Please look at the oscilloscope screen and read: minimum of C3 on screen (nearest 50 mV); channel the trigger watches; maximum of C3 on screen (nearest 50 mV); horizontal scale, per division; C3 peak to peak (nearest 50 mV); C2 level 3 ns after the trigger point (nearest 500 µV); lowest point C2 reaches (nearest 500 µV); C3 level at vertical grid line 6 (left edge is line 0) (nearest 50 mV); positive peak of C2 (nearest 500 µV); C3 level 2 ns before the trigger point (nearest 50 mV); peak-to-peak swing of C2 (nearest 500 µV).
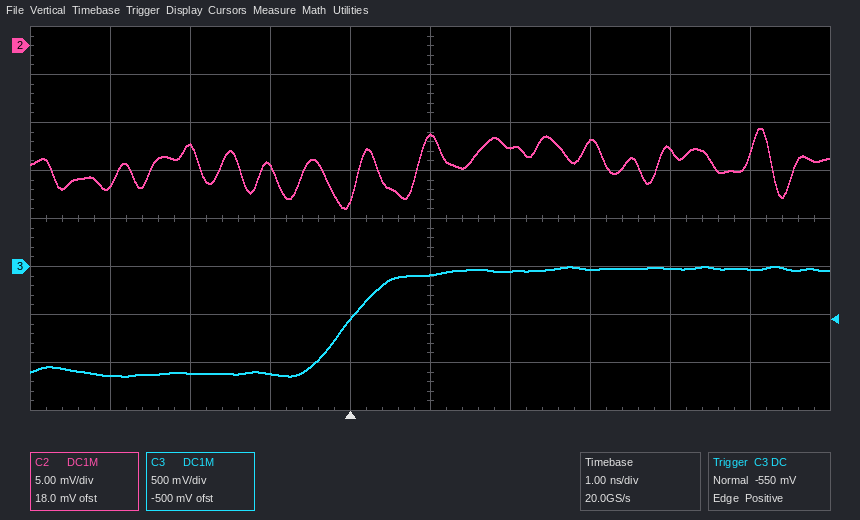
-1.15 V
C3
0 mV
1 ns
1.15 V
-10.0 mV
-17.0 mV
-50 mV
-8.5 mV
-1.10 V
8.5 mV
